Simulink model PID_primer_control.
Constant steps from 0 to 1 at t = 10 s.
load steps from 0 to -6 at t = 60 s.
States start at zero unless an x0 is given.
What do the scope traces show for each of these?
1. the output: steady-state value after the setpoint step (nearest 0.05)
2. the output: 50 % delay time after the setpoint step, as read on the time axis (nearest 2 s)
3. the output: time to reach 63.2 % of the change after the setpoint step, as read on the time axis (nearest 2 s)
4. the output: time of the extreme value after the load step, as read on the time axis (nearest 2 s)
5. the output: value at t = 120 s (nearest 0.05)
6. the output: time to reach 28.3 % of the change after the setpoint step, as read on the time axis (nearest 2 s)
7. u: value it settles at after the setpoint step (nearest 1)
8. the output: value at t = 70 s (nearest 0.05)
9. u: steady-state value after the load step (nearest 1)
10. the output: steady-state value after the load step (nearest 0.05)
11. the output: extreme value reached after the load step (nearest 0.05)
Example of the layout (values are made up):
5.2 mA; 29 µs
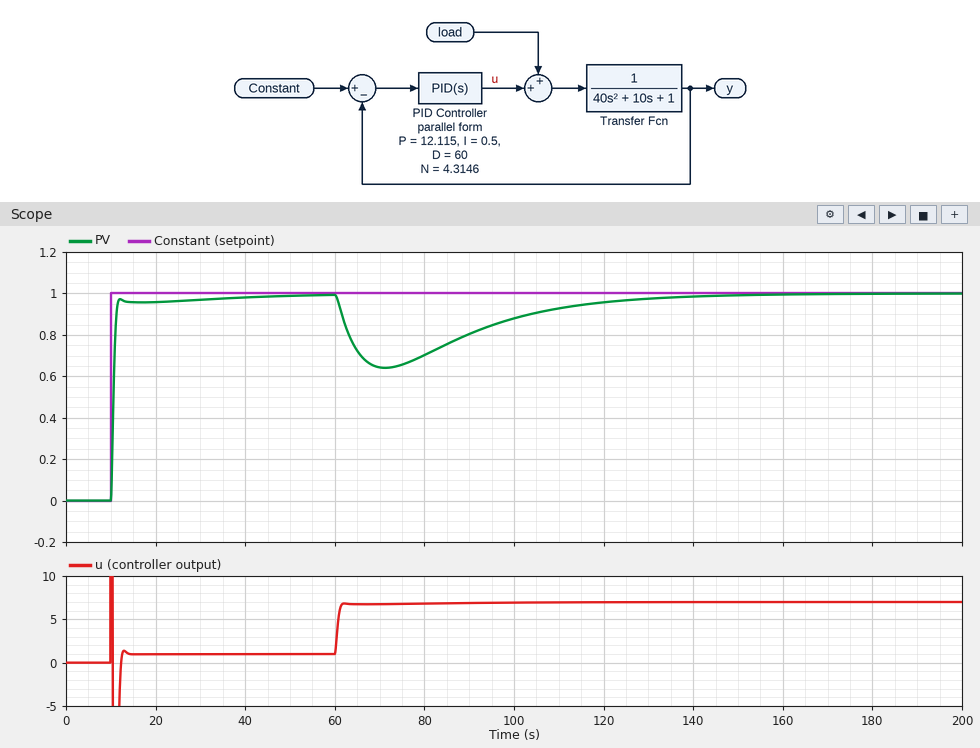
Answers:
1.00; 10 s; 10 s; 72 s; 0.95; 10 s; 1; 0.65; 7; 1.00; 0.65
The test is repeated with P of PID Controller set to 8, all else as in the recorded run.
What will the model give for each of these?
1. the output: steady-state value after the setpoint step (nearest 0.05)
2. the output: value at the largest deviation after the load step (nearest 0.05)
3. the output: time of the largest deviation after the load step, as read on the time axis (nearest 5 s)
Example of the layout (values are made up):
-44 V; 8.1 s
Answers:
1.00; 0.55; 75 s
